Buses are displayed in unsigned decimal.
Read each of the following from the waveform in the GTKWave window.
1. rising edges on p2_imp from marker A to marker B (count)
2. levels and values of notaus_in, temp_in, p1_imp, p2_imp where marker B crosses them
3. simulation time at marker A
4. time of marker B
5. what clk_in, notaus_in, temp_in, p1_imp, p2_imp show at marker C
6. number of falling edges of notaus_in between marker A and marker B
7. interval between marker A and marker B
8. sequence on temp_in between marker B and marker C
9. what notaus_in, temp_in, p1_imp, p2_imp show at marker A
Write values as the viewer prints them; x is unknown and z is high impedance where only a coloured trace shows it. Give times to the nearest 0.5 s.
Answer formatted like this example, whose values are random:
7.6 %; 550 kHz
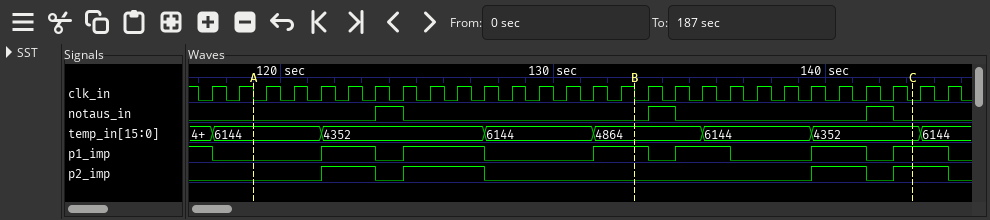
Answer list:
2; notaus_in=0, temp_in=4864, p1_imp=1, p2_imp=0; 119 s; 133 s; clk_in=0, notaus_in=0, temp_in=4352, p1_imp=1, p2_imp=1; 1; 14 s; 4864, 6144, 4352; notaus_in=0, temp_in=6144, p1_imp=0, p2_imp=0
